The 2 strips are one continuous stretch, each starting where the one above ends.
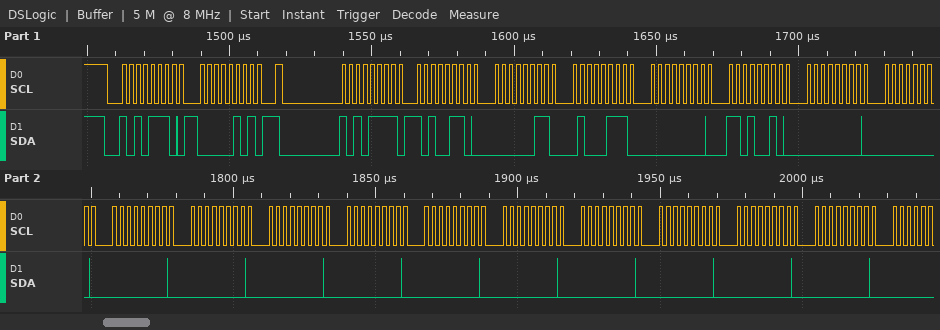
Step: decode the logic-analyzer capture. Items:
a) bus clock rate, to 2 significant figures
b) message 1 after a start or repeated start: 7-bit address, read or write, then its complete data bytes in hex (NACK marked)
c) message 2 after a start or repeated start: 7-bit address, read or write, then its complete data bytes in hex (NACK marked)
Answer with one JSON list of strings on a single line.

["400 kHz", "0x57 write: 05", "0x57 read: A6 03 47 00 D2 00 00 00 00 00 00 00 00 00 00 00 00"]
